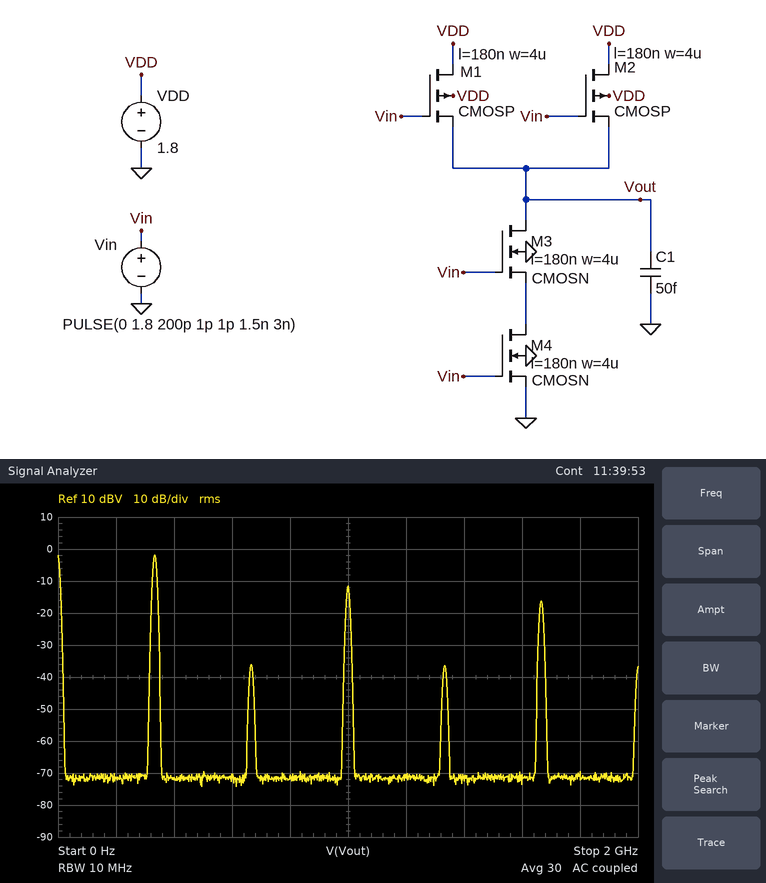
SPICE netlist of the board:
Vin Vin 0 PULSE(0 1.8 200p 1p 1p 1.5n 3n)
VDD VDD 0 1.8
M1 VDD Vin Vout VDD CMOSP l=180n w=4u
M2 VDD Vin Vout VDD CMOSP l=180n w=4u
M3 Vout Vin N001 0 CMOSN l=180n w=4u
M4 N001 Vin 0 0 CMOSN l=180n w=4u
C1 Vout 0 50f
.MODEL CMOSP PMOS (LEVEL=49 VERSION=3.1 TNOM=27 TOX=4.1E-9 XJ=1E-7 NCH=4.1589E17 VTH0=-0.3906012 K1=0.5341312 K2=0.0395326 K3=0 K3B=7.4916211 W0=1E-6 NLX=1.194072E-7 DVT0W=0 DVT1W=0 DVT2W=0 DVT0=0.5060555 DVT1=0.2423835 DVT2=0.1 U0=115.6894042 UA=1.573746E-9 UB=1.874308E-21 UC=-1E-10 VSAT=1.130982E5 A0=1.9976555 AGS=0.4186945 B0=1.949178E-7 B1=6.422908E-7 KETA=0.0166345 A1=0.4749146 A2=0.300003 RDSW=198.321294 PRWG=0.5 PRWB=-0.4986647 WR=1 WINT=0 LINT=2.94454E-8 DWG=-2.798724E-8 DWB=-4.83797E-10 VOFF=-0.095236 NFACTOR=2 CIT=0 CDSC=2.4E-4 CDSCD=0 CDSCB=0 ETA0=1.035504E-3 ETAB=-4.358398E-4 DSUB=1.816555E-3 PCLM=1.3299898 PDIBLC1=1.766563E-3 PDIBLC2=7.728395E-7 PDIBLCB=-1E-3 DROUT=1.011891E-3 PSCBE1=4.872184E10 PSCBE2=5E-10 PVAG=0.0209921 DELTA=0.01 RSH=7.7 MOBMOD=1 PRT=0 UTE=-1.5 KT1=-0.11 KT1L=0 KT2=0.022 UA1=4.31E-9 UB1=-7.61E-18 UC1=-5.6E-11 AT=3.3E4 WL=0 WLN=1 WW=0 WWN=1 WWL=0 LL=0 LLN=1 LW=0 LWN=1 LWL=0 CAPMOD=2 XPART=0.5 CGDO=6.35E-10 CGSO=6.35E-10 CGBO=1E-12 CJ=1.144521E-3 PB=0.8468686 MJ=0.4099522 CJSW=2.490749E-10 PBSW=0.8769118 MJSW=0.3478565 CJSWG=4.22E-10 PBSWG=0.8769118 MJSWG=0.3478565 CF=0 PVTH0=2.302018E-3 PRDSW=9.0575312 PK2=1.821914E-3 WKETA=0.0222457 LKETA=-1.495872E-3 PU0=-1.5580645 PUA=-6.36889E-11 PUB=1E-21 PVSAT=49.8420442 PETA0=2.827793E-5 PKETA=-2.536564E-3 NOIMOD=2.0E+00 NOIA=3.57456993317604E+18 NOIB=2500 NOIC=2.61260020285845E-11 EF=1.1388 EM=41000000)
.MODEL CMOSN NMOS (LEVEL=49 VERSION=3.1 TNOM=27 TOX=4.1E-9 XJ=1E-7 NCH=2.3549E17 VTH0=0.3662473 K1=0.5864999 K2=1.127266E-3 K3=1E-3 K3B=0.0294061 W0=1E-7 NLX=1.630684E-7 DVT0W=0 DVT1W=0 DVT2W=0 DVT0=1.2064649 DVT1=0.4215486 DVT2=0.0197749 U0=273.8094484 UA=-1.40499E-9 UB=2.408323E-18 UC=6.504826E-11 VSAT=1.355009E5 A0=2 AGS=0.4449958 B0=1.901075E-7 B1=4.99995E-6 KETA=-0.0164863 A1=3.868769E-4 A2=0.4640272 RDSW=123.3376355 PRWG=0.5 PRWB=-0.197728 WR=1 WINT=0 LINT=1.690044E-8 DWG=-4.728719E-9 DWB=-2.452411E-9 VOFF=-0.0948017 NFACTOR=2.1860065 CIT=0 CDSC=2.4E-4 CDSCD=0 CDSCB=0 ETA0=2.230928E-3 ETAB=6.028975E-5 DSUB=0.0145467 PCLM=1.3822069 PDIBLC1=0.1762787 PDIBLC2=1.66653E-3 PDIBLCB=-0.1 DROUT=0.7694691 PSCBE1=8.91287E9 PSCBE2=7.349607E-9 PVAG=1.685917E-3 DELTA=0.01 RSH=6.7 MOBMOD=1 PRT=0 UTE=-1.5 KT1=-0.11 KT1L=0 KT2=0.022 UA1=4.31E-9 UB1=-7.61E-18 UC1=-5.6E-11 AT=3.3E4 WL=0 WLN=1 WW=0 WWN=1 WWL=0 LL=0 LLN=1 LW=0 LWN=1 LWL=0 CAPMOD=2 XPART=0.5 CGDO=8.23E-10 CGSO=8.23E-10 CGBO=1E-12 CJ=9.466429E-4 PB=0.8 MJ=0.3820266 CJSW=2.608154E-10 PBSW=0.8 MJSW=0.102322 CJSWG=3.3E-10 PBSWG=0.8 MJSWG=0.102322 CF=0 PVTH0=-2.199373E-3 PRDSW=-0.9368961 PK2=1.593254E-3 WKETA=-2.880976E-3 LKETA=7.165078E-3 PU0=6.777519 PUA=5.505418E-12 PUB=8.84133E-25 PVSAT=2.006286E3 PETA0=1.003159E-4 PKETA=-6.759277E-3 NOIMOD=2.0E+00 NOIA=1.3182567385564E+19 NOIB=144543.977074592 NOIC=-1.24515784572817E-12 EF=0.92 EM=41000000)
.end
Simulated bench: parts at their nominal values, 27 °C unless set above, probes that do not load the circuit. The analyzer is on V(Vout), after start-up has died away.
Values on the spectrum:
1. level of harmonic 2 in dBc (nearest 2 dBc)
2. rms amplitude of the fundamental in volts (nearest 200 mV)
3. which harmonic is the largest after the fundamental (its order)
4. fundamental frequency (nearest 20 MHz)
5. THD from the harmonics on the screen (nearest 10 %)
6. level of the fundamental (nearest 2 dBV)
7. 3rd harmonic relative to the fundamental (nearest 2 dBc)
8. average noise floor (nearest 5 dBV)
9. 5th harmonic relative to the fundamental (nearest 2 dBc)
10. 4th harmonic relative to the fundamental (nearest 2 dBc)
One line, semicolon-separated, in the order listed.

-34 dBc; 800 mV; 3; 340 MHz; 40 %; -2 dBV; -10 dBc; -70 dBV; -14 dBc; -34 dBc
